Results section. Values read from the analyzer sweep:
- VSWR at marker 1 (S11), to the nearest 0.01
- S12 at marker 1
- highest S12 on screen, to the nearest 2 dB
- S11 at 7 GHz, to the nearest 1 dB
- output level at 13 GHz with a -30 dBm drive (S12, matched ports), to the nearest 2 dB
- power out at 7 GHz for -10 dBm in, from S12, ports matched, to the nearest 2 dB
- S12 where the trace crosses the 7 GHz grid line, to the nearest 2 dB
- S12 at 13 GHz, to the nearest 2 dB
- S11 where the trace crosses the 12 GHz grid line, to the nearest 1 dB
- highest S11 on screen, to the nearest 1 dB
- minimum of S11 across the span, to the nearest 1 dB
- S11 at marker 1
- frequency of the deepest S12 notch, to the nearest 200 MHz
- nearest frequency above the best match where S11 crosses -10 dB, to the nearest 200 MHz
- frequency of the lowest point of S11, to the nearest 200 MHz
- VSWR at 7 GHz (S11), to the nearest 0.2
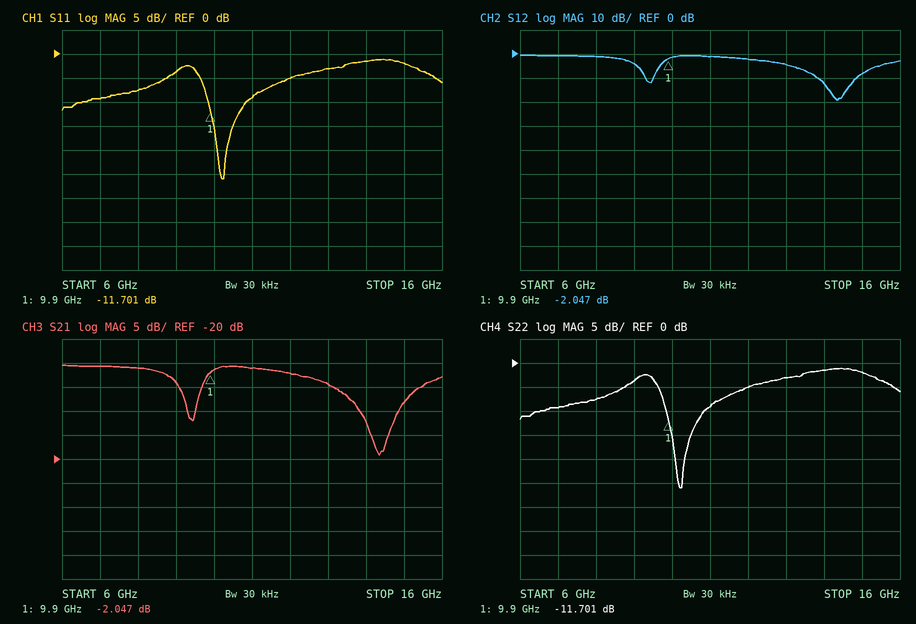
1.70
-2.047 dB
0 dB
-9 dB
-34 dBm
-10 dBm
0 dB
-4 dB
-5 dB
-1 dB
-26 dB
-11.701 dB
14.4 GHz
10.8 GHz
10.2 GHz
2.0
